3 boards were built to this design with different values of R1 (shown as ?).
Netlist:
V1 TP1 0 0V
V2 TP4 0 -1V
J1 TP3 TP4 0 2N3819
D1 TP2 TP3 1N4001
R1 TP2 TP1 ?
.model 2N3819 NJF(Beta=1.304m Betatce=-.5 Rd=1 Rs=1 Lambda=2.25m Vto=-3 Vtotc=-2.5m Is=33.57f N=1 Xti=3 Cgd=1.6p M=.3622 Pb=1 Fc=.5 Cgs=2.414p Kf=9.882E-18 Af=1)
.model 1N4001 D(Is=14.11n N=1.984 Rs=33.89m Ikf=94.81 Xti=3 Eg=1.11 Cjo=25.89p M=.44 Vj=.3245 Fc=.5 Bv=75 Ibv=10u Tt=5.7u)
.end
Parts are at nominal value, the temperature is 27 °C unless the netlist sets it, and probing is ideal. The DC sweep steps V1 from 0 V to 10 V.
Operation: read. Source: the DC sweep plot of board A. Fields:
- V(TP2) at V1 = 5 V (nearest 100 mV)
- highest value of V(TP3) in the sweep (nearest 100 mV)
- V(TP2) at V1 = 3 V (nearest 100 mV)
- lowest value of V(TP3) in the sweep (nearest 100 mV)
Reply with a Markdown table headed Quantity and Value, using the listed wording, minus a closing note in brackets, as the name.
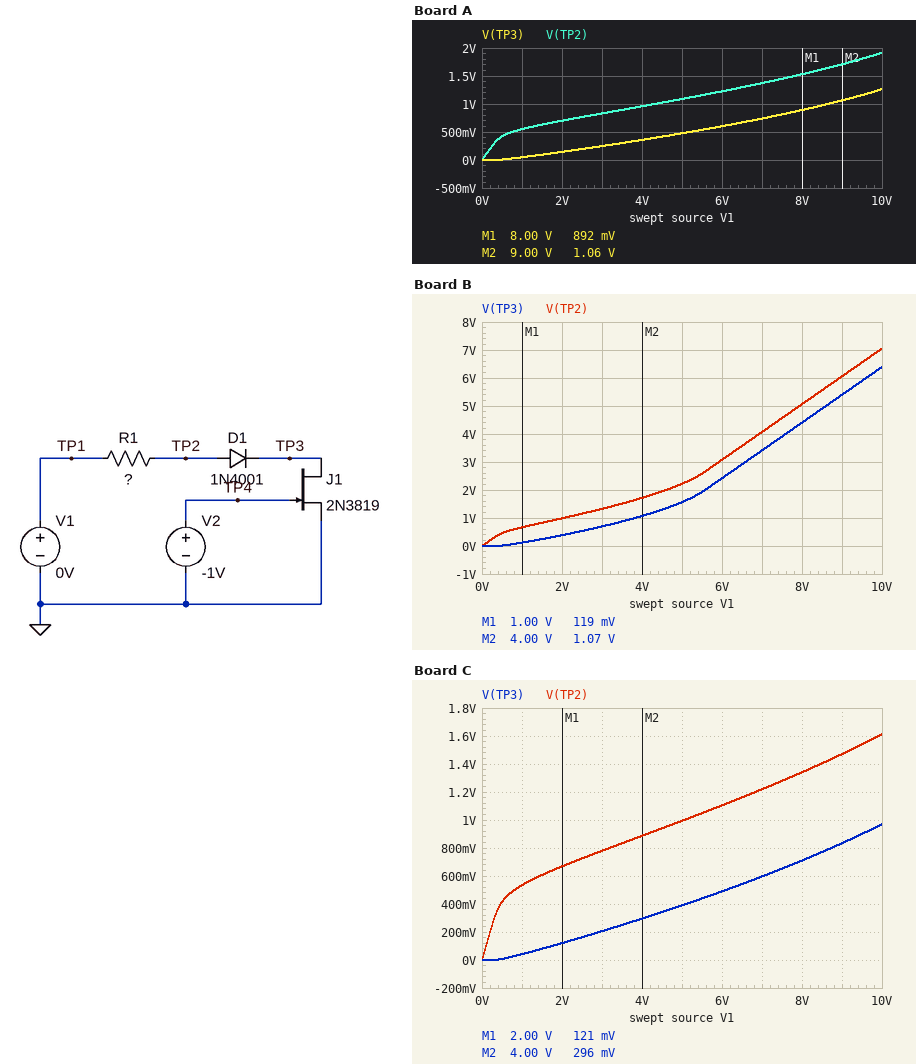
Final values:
| Quantity | Value |
|---|---|
| V(TP2) at V1 = 5 V | 1.1 V |
| highest value of V(TP3) in the sweep | 1.3 V |
| V(TP2) at V1 = 3 V | 800 mV |
| lowest value of V(TP3) in the sweep | 0 V |
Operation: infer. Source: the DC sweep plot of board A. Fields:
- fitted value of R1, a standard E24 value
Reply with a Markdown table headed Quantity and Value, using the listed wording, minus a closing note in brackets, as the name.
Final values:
| Quantity | Value |
|---|---|
| fitted value of R1, a standard E24 value | 1.8 kΩ |
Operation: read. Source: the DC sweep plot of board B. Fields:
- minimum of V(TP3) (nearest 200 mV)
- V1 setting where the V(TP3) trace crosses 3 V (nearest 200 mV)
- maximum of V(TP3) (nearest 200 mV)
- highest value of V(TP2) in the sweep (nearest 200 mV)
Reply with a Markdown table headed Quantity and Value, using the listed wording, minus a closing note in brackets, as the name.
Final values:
| Quantity | Value |
|---|---|
| minimum of V(TP3) | 0 V |
| V1 setting where the V(TP3) trace crosses 3 V | 6.6 V |
| maximum of V(TP3) | 6.4 V |
| highest value of V(TP2) in the sweep | 7.0 V |
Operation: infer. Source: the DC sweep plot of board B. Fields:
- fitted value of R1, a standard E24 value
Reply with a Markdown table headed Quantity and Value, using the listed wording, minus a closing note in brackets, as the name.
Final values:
| Quantity | Value |
|---|---|
| fitted value of R1, a standard E24 value | 560 Ω |
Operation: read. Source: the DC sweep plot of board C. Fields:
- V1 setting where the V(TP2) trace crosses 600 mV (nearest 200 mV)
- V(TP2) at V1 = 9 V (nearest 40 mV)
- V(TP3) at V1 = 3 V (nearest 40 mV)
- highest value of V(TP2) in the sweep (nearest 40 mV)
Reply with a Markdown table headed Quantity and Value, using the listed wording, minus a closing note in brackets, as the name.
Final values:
| Quantity | Value |
|---|---|
| V1 setting where the V(TP2) trace crosses 600 mV | 1.4 V |
| V(TP2) at V1 = 9 V | 1.48 V |
| V(TP3) at V1 = 3 V | 200 mV |
| highest value of V(TP2) in the sweep | 1.60 V |
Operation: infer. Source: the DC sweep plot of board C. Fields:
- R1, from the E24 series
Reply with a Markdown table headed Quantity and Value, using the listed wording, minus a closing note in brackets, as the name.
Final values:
| Quantity | Value |
|---|---|
| R1, from the E24 series | 2.2 kΩ |
